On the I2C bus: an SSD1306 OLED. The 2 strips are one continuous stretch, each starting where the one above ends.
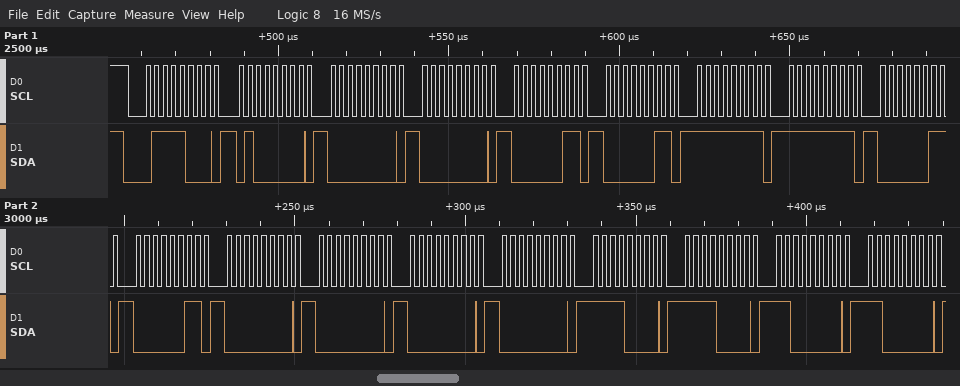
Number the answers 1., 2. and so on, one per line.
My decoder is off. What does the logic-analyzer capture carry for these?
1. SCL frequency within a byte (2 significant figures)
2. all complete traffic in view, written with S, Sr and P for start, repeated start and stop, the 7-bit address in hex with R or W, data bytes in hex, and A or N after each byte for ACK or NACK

1. 400 kHz
2. S 3CW A 40 A 00 A 00 A 03 A 03 A FF A FF A 03 A 03 A 00 A 00 A 00 A 00 A F0 A F0 A C0 A C0 A
